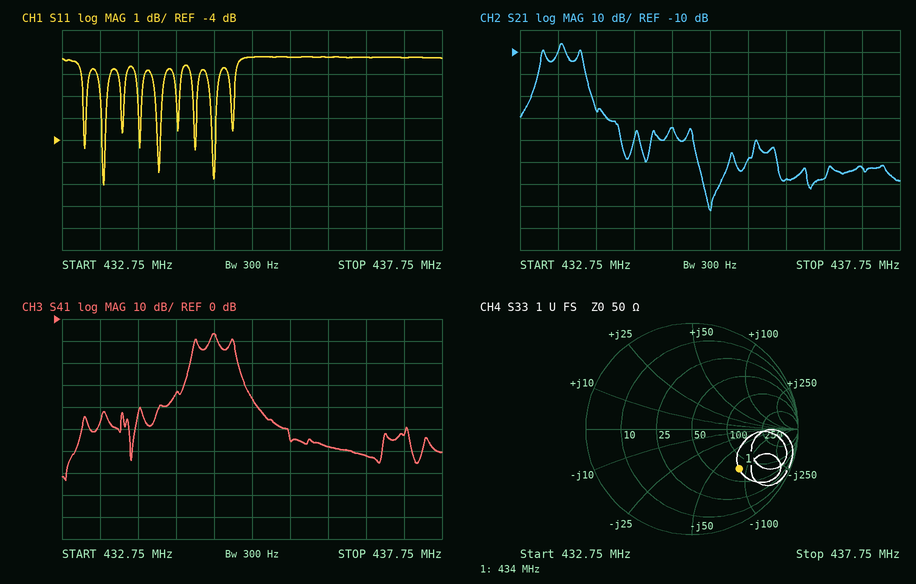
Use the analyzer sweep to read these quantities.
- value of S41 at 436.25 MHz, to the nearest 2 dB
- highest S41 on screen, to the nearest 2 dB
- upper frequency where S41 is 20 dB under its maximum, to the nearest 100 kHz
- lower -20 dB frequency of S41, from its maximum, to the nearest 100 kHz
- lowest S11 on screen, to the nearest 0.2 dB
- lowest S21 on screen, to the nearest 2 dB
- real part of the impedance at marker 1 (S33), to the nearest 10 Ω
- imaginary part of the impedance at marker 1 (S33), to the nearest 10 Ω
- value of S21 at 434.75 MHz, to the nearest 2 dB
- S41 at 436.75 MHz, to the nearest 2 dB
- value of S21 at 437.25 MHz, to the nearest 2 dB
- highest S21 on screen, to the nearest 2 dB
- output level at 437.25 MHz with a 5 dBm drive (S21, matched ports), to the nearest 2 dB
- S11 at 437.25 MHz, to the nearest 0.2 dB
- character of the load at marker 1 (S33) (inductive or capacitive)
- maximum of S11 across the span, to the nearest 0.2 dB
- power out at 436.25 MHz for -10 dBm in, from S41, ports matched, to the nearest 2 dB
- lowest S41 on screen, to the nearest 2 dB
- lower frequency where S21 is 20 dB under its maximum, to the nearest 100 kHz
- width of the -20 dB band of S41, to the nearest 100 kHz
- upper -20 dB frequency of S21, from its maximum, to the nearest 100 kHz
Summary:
-58 dB
-6 dB
435.1 MHz
434.4 MHz
-6.0 dB
-82 dB
70 Ω
-80 Ω
-44 dB
-62 dB
-62 dB
-6 dB
-58 dBm
-0.2 dB
capacitive
-0.2 dB
-68 dBm
-74 dB
432.9 MHz
700 kHz
433.7 MHz
